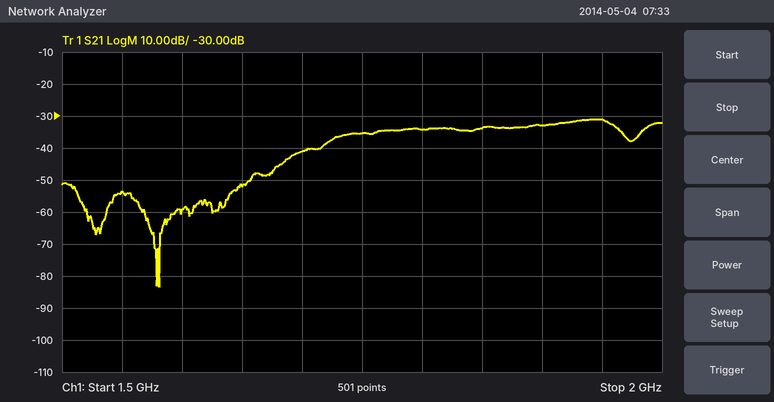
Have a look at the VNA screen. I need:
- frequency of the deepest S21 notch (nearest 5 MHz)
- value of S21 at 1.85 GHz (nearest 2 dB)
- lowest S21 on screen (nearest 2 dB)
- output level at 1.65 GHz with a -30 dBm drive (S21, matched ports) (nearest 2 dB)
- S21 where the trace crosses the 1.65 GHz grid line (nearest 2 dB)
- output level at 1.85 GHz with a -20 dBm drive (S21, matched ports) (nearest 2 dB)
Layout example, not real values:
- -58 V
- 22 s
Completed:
- 1.580 GHz
- -34 dB
- -84 dB
- -82 dBm
- -52 dB
- -54 dBm
